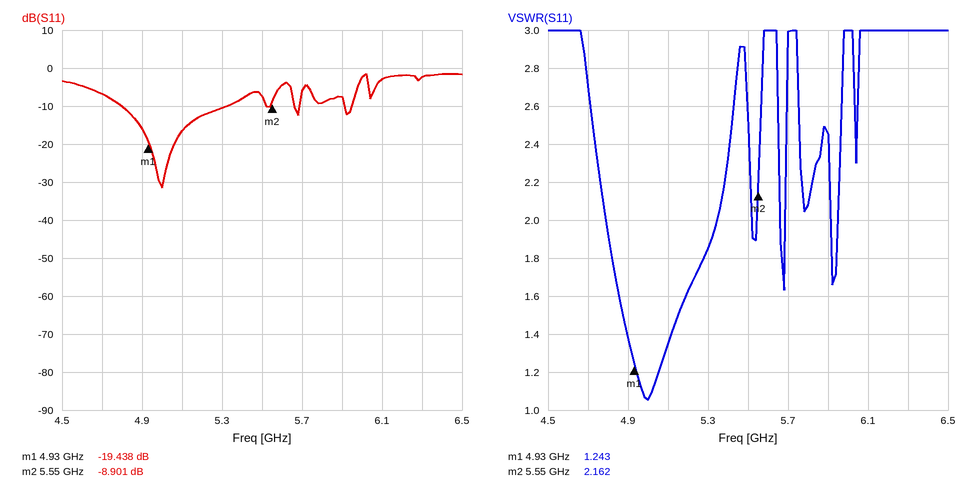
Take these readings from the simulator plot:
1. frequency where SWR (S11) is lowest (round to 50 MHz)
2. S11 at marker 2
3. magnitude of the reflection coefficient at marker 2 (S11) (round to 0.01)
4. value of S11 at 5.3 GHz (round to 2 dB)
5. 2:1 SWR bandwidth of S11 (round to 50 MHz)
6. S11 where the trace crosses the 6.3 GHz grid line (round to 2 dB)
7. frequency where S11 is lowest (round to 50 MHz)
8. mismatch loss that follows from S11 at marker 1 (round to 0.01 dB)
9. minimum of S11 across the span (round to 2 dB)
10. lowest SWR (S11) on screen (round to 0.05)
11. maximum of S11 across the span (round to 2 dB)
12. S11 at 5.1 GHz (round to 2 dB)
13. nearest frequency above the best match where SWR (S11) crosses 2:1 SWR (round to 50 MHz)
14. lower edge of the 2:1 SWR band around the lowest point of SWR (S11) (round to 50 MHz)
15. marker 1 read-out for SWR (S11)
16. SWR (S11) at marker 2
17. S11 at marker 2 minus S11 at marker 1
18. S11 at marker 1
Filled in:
5.00 GHz
-8.901 dB
0.36
-10 dB
550 MHz
-2 dB
5.00 GHz
0.05 dB
-32 dB
1.05
-2 dB
-16 dB
5.35 GHz
4.80 GHz
1.243
2.162
10.537 dB
-19.438 dB
